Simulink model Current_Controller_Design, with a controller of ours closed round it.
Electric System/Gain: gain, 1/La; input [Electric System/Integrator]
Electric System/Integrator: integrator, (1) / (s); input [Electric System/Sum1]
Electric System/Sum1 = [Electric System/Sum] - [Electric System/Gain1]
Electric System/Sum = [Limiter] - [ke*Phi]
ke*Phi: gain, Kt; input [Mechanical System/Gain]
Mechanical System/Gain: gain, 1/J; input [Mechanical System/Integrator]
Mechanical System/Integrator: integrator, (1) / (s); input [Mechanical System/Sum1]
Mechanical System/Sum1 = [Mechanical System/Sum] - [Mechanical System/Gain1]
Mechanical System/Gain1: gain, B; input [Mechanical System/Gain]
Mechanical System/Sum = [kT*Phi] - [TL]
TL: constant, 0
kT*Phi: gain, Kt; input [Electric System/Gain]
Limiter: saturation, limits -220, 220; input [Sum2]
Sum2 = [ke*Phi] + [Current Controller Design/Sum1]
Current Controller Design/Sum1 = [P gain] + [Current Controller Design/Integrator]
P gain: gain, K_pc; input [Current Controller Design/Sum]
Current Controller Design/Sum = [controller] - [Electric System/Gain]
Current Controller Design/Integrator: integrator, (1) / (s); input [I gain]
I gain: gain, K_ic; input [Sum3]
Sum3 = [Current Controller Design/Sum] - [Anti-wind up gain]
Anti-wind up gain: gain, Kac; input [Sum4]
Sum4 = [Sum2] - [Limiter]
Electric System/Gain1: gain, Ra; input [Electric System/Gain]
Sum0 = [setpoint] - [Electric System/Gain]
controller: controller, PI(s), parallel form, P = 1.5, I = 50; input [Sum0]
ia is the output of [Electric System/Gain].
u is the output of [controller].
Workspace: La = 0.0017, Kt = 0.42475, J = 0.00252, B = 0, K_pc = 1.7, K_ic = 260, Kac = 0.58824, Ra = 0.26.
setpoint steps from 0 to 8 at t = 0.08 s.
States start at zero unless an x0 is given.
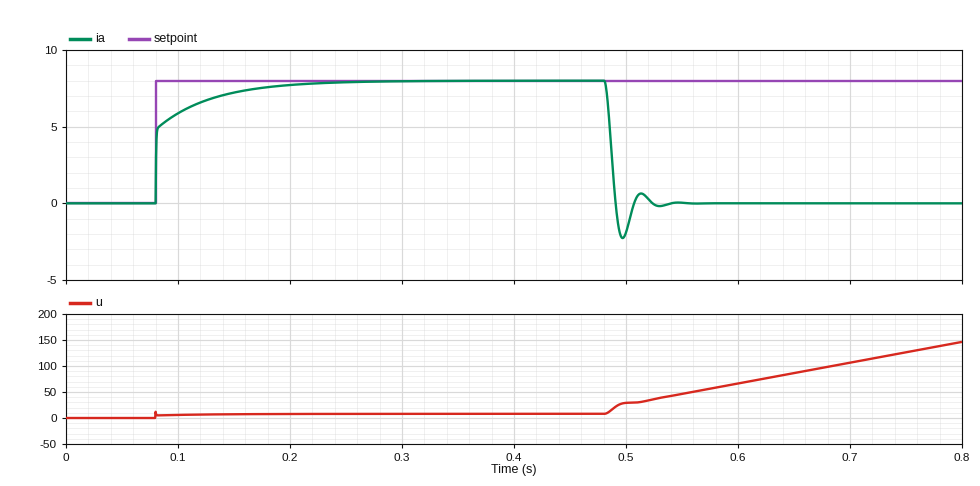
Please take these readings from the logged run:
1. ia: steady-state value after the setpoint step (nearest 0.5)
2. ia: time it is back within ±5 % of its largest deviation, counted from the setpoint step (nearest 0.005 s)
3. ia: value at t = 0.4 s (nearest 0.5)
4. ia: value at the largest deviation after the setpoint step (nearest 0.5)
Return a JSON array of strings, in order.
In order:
["0.0", "0.440 s", "8.0", "8.0"]
